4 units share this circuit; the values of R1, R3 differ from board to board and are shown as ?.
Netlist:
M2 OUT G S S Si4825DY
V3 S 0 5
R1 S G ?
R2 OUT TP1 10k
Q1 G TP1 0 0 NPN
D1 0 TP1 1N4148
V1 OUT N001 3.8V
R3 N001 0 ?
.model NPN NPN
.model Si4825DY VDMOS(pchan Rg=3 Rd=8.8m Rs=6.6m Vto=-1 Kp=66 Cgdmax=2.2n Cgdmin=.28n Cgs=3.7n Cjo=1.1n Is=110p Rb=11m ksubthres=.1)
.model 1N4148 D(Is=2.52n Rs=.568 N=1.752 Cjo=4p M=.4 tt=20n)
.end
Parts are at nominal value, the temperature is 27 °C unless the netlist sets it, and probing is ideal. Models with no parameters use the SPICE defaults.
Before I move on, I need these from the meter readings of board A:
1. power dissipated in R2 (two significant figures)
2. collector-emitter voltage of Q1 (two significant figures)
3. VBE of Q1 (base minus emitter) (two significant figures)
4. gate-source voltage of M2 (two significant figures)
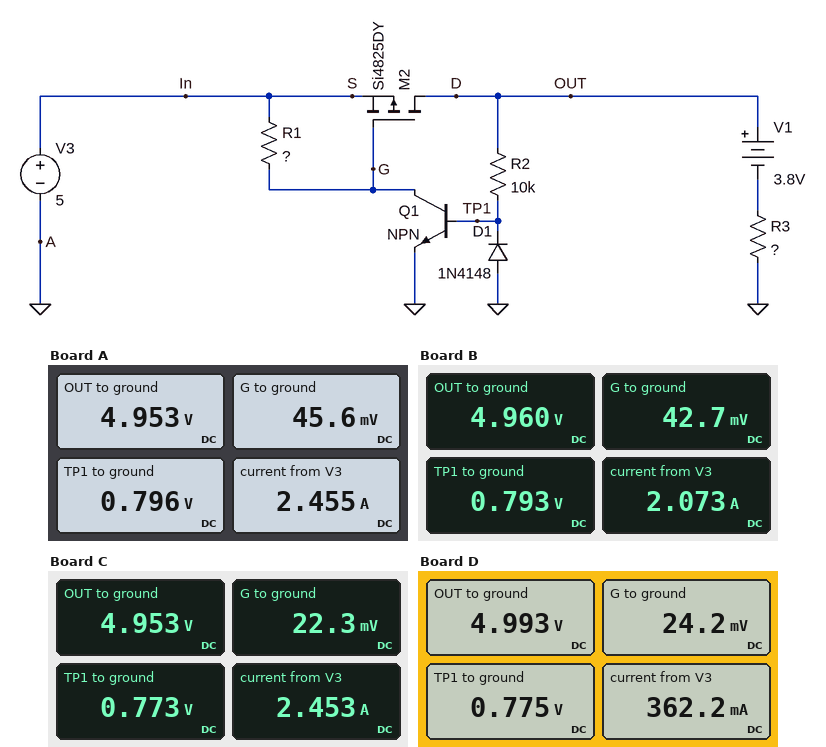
1.7 mW
46 mV
800 mV
-5.0 V
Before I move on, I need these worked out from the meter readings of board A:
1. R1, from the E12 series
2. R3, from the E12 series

3.3 kΩ
0.47 Ω
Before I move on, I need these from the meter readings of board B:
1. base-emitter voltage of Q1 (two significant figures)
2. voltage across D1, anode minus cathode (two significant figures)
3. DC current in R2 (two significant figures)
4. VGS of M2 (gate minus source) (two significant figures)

790 mV
-790 mV
420 µA
-5.0 V
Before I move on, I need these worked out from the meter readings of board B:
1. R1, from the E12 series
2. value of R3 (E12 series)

3.9 kΩ
0.56 Ω
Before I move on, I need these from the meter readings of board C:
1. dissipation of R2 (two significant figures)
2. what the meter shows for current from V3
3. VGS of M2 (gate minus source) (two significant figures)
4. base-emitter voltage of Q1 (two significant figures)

1.7 mW
2.453 A
-5.0 V
770 mV
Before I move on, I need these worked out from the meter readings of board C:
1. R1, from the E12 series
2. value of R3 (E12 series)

33 kΩ
0.47 Ω
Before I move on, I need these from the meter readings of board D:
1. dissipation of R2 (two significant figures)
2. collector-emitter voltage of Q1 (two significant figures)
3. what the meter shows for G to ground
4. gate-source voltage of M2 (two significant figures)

1.8 mW
24 mV
24.2 mV
-5.0 V
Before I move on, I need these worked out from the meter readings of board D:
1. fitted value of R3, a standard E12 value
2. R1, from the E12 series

3.3 Ω
22 kΩ
